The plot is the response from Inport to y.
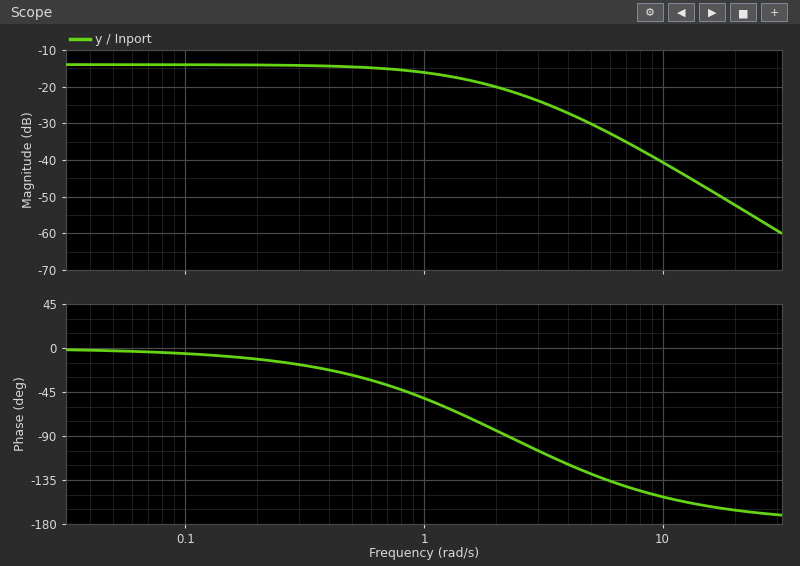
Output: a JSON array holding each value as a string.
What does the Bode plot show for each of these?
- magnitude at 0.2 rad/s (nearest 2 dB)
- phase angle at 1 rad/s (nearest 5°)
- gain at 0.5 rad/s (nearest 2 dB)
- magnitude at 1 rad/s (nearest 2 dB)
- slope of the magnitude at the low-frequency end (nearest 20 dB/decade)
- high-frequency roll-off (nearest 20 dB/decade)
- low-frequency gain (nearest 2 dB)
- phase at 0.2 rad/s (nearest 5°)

["-14 dB", "-50°", "-14 dB", "-16 dB", "0 dB/decade", "-40 dB/decade", "-14 dB", "-10°"]
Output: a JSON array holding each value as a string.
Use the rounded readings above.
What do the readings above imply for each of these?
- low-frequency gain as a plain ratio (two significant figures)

["0.20"]
